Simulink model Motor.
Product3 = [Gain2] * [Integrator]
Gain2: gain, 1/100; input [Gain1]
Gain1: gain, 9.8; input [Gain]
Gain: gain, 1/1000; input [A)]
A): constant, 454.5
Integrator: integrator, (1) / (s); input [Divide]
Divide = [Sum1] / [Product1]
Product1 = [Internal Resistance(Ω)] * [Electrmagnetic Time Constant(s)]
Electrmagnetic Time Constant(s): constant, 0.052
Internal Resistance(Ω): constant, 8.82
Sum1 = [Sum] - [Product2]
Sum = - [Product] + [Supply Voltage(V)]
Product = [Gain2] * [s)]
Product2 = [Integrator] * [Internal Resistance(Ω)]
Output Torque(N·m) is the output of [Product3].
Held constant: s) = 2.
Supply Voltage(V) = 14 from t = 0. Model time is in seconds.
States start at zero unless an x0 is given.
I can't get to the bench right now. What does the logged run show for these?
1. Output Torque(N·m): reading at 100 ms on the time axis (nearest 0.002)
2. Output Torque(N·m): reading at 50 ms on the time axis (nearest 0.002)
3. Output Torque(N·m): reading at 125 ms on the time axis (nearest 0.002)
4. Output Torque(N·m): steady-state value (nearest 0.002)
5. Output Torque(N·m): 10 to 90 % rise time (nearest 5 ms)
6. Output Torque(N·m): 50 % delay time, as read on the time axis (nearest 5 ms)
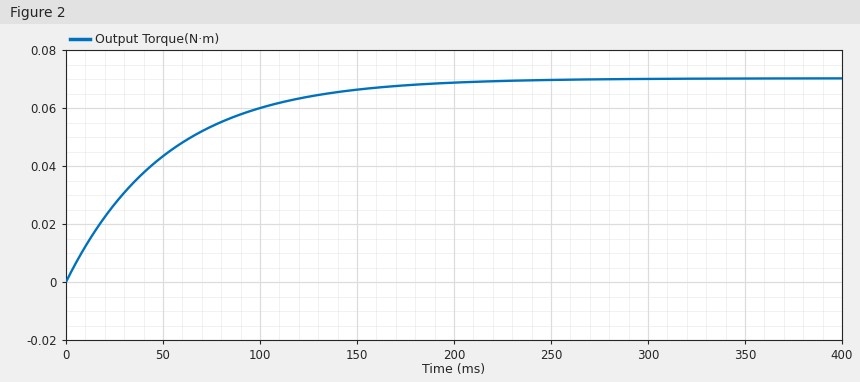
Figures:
0.060
0.044
0.064
0.070
115 ms
35 ms
